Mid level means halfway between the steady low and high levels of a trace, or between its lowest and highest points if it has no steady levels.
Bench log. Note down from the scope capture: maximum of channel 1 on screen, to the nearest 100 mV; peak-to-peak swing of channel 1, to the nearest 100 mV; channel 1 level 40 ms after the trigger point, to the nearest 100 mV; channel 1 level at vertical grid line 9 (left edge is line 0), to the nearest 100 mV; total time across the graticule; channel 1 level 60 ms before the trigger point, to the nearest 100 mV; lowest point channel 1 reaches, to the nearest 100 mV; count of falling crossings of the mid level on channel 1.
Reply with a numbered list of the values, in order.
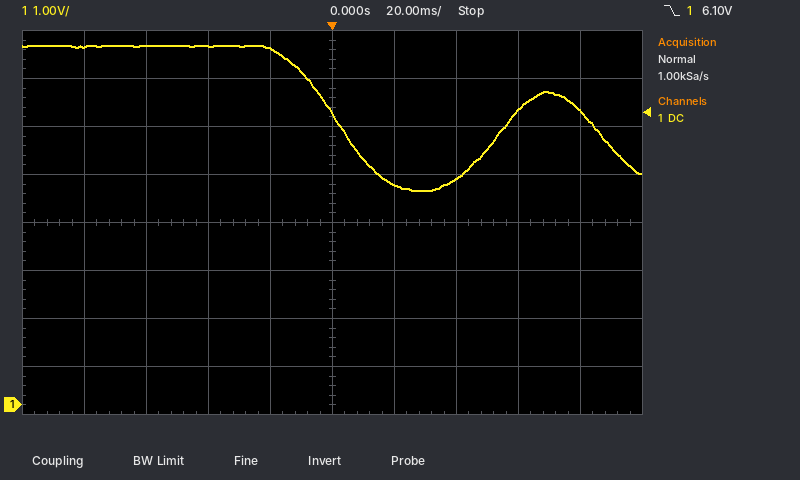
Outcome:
1. 7.5 V
2. 3.0 V
3. 4.7 V
4. 6.1 V
5. 200 ms
6. 7.5 V
7. 4.5 V
8. 2
